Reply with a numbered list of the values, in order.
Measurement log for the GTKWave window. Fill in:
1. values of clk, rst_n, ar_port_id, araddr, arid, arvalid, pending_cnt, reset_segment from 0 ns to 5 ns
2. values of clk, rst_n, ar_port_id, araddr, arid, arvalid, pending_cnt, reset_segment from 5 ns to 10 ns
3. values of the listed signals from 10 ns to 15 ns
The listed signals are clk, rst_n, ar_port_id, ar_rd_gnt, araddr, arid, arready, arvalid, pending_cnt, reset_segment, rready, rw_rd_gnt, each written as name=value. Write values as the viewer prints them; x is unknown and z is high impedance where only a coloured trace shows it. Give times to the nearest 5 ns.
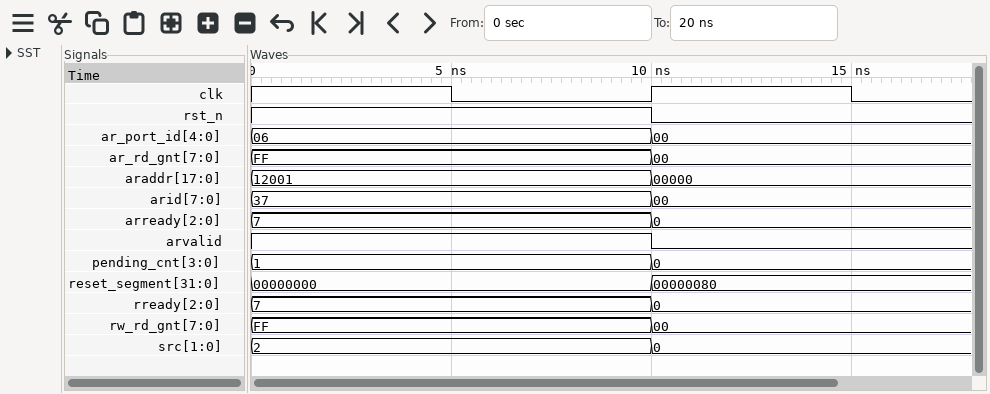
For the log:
1. clk=1, rst_n=1, ar_port_id=06, araddr=12001, arid=37, arvalid=1, pending_cnt=1, reset_segment=00000000
2. clk=0, rst_n=1, ar_port_id=06, araddr=12001, arid=37, arvalid=1, pending_cnt=1, reset_segment=00000000
3. clk=1, rst_n=0, ar_port_id=00, ar_rd_gnt=00, araddr=00000, arid=00, arready=0, arvalid=0, pending_cnt=0, reset_segment=00000080, rready=0, rw_rd_gnt=00
